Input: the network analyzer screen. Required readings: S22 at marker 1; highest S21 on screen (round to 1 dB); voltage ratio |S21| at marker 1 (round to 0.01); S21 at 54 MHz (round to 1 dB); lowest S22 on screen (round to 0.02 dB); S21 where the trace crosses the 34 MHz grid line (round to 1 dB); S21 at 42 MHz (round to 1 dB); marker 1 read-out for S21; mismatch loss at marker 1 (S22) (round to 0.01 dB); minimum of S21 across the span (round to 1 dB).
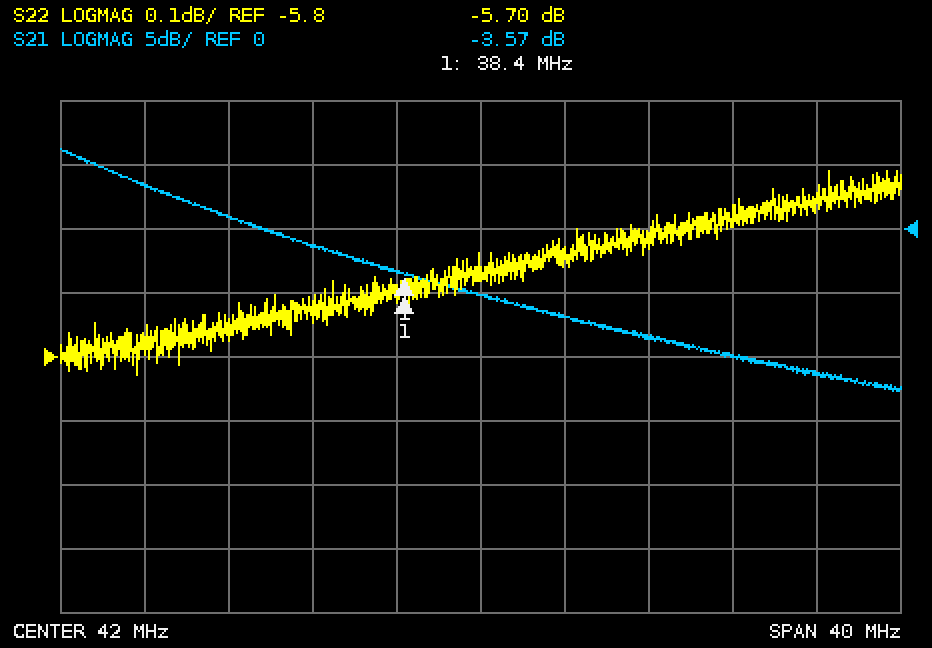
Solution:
-5.70 dB
6 dB
0.66
-10 dB
-5.82 dB
-1 dB
-5 dB
-3.57 dB
1.36 dB
-13 dB
